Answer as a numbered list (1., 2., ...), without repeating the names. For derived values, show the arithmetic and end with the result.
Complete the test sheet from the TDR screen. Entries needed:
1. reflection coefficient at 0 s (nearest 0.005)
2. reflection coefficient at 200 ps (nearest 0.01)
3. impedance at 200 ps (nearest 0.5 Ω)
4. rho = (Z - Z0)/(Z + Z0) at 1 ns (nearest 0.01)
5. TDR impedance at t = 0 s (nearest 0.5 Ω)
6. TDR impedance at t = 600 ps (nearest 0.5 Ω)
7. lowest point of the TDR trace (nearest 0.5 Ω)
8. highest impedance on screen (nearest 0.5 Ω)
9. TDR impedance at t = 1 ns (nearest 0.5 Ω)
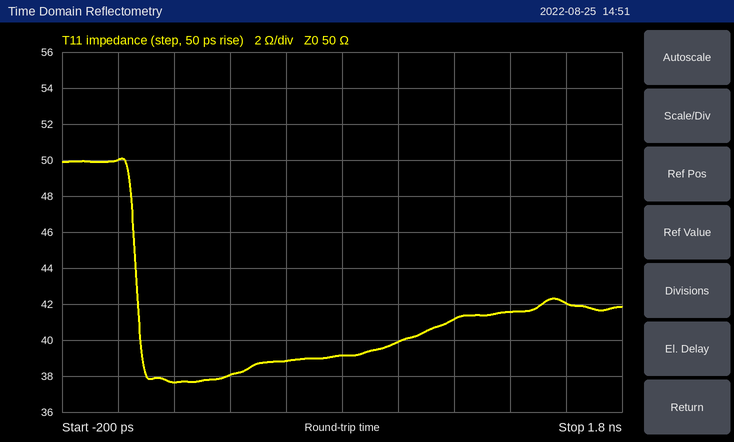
1. (50 − 50)/(50 + 50) ≈ 0.000
2. (37.5 − 50)/(37.5 + 50) ≈ -0.14
3. 37.5 Ω
4. (40 − 50)/(40 + 50) ≈ -0.11
5. 50.0 Ω
6. 39.0 Ω
7. 37.5 Ω
8. 50.0 Ω
9. 40.0 Ω
